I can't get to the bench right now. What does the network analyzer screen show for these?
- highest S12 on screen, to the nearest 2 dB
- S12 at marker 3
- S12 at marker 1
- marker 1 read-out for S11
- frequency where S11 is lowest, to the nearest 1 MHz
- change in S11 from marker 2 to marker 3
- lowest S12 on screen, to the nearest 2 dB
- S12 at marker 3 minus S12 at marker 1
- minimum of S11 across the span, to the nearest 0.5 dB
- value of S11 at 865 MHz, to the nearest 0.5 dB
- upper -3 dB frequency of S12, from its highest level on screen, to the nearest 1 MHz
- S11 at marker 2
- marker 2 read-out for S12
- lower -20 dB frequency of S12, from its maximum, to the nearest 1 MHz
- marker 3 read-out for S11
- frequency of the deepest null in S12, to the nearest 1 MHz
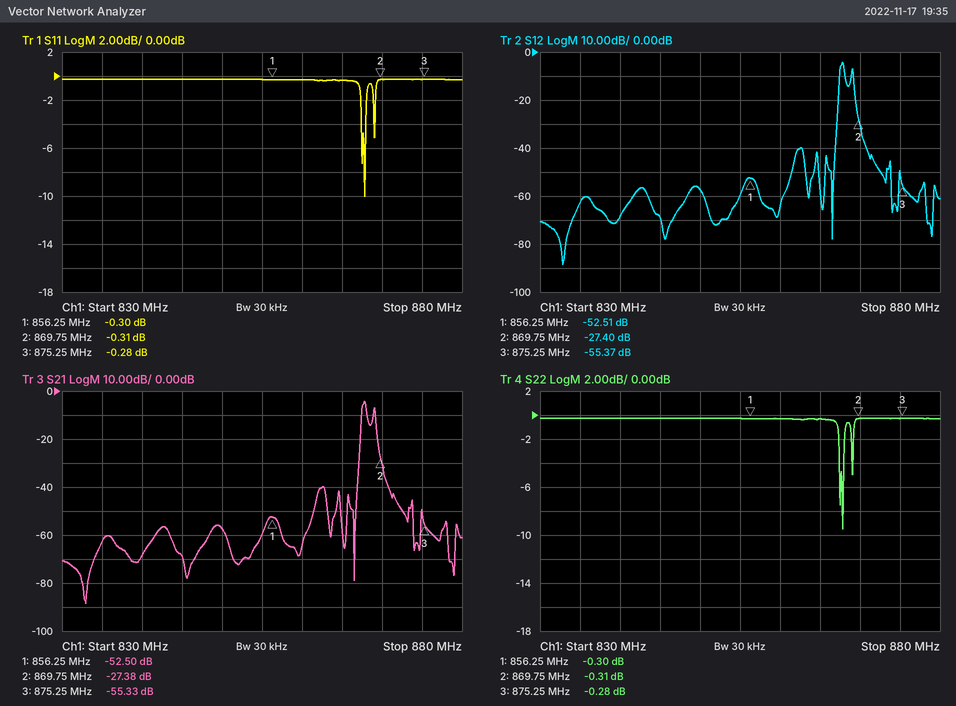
-4 dB
-55.37 dB
-52.51 dB
-0.30 dB
868 MHz
0.03 dB
-88 dB
-2.86 dB
-10.0 dB
-0.5 dB
868 MHz
-0.31 dB
-27.40 dB
867 MHz
-0.28 dB
833 MHz
